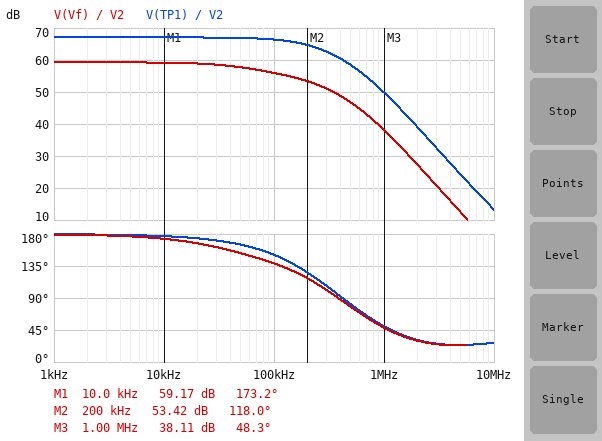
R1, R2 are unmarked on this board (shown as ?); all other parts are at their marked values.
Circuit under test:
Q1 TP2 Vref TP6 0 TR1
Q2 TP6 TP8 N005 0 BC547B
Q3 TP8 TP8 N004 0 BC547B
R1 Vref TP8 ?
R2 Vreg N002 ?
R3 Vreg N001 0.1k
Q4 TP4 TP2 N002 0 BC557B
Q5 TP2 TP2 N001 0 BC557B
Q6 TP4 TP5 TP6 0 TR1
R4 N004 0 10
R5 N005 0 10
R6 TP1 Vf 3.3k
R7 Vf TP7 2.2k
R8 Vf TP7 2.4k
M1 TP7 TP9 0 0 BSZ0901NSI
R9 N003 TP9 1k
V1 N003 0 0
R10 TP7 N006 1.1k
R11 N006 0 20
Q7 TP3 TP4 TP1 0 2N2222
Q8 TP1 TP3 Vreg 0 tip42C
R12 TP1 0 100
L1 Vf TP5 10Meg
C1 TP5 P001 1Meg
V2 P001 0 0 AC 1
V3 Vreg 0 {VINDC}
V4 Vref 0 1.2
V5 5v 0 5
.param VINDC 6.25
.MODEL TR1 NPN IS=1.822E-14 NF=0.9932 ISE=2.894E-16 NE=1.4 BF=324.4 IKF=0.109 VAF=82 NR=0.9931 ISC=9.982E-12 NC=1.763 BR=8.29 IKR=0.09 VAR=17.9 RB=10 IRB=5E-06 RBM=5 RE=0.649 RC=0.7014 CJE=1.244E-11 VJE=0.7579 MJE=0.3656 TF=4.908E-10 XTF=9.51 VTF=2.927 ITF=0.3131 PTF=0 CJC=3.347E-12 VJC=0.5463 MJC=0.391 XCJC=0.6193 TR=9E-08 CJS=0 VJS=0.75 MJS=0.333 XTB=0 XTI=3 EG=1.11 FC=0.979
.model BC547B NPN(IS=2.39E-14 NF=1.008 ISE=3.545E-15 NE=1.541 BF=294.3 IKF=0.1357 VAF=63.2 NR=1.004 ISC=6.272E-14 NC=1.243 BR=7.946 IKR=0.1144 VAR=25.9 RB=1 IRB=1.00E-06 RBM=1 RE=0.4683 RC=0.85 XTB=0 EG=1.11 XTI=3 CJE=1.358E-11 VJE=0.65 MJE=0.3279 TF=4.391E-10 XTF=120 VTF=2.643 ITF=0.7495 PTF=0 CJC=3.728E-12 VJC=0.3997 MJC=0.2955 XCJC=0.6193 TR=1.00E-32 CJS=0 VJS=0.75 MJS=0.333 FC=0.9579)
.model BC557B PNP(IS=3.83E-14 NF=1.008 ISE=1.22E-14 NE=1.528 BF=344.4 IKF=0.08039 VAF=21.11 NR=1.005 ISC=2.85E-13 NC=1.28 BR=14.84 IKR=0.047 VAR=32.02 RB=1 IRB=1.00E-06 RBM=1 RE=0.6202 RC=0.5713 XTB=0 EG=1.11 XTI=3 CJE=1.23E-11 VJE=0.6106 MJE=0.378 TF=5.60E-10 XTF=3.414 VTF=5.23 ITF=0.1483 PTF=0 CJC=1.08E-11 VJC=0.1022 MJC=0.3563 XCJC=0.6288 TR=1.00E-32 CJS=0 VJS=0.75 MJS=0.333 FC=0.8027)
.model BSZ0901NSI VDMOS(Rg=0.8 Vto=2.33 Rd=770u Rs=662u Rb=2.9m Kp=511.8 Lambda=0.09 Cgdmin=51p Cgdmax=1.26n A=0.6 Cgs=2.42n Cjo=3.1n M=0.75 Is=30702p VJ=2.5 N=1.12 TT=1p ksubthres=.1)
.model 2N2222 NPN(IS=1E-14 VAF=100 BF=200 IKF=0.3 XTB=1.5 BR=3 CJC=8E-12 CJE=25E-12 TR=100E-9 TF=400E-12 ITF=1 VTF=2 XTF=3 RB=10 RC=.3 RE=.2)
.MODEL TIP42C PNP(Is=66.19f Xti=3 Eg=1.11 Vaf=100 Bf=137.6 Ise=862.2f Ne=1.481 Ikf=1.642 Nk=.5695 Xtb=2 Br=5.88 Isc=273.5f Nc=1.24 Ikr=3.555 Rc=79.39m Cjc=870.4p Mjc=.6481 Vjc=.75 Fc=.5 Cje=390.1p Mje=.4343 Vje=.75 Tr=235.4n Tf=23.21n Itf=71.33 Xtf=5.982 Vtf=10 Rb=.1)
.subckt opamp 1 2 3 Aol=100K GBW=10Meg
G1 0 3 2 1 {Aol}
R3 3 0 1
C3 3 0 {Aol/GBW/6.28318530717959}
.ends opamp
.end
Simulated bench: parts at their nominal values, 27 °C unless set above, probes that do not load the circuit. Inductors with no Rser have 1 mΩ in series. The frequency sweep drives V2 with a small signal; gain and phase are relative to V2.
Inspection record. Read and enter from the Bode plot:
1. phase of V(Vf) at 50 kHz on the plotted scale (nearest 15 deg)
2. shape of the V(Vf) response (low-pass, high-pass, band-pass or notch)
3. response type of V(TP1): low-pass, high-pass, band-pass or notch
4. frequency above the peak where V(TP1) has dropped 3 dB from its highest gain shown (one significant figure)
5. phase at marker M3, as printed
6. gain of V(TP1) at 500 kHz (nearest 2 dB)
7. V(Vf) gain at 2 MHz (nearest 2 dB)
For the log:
150 deg
low-pass
low-pass
200 kHz
48.3 deg
58 dB
28 dB
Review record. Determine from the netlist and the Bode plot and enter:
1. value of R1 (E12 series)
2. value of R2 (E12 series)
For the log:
120 Ω
220 Ω
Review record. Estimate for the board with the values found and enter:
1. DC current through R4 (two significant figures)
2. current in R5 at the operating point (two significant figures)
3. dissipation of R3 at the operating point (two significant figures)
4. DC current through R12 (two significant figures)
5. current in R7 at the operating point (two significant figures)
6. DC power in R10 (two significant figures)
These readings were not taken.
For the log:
4.0 mA
4.0 mA
710 µW
29 mA
270 µA
300 µW
